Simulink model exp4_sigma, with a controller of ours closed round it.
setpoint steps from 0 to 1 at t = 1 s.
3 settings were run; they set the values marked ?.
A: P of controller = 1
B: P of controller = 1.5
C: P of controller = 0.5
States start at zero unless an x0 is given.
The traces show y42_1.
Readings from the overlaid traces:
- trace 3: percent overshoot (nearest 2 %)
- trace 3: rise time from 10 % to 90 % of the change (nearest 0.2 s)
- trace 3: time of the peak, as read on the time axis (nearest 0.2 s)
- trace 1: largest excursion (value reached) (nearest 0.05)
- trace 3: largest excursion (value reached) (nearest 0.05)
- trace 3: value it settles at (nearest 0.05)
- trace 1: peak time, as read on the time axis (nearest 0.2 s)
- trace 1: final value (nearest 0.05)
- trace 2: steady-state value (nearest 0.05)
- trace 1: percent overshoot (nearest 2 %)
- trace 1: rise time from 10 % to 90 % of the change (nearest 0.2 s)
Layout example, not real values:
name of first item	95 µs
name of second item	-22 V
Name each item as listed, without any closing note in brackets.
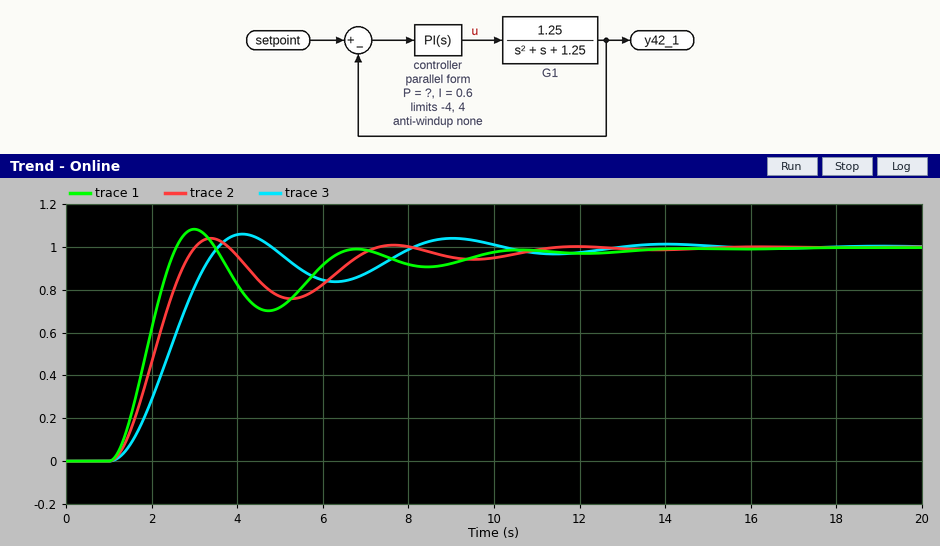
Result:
trace 3: percent overshoot	6 %
trace 3: rise time from 10 % to 90 % of the change	1.6 s
trace 3: time of the peak, as read on the time axis	4.2 s
trace 1: largest excursion (value reached)	1.10
trace 3: largest excursion (value reached)	1.05
trace 3: value it settles at	1.00
trace 1: peak time, as read on the time axis	3.0 s
trace 1: final value	1.00
trace 2: steady-state value	1.00
trace 1: percent overshoot	8 %
trace 1: rise time from 10 % to 90 % of the change	1.0 s
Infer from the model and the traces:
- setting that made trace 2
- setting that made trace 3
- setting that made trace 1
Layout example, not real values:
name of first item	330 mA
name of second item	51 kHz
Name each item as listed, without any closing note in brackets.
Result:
setting that made trace 2	A
setting that made trace 3	C
setting that made trace 1	B
